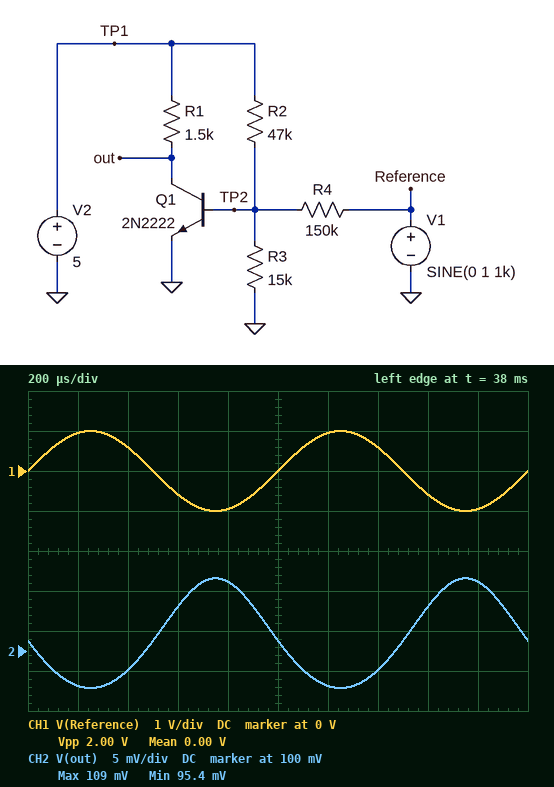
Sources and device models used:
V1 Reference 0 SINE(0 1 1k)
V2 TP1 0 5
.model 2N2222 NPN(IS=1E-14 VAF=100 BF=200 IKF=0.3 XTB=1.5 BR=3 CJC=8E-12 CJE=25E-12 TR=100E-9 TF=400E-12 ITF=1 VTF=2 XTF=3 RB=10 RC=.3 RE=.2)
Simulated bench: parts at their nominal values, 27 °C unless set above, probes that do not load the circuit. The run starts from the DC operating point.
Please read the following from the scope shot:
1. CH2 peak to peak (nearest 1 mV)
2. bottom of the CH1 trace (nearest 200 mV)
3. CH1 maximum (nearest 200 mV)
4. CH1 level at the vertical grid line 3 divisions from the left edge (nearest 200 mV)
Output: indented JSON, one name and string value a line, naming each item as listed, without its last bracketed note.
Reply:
{
  "CH2 peak to peak": "14 mV",
  "bottom of the CH1 trace": "-1.0 V",
  "CH1 maximum": "1.0 V",
  "CH1 level at the vertical grid line 3 divisions from the left edge": "-600 mV"
}
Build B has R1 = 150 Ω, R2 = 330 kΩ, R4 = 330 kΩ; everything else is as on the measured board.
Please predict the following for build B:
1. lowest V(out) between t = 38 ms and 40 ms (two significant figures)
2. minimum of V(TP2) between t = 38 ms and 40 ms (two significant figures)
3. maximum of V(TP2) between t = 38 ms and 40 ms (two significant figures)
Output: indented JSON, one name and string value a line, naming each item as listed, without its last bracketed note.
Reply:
{
  "lowest V(out) between t = 38 ms and 40 ms": "5.0 V",
  "minimum of V(TP2) between t = 38 ms and 40 ms": "170 mV",
  "maximum of V(TP2) between t = 38 ms and 40 ms": "250 mV"
}
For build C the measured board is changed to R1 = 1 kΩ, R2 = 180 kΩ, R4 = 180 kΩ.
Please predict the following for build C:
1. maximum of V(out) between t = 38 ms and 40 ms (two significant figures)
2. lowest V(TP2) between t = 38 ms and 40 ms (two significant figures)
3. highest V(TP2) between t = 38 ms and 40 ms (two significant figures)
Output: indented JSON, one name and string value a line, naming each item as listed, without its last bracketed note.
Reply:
{
  "maximum of V(out) between t = 38 ms and 40 ms": "5.0 V",
  "lowest V(TP2) between t = 38 ms and 40 ms": "290 mV",
  "highest V(TP2) between t = 38 ms and 40 ms": "430 mV"
}
